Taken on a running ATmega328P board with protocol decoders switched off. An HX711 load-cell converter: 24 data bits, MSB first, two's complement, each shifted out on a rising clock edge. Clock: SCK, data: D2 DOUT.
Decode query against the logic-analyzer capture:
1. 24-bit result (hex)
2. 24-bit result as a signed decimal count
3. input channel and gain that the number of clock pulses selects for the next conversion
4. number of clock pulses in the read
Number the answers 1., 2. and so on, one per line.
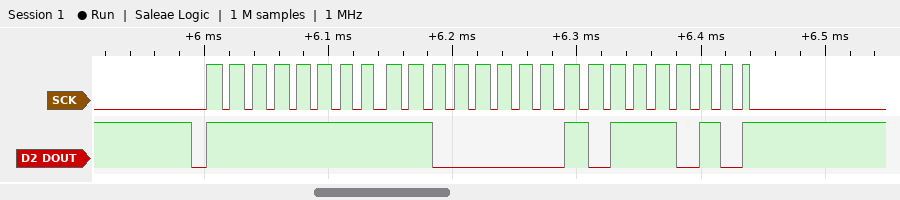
1. 0xFFC0BA
2. -16198
3. channel A, gain 128
4. 25
